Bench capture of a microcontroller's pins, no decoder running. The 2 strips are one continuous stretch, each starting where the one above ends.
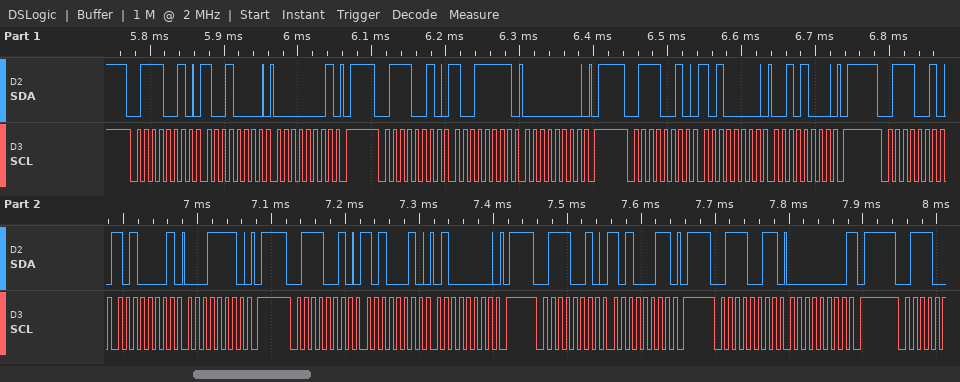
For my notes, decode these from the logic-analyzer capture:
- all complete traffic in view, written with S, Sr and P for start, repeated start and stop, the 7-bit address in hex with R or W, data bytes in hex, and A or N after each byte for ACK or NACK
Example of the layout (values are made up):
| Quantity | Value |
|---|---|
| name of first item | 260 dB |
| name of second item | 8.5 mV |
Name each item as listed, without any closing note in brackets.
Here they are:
| Quantity | Value |
|---|---|
| all complete traffic in view, written with S, Sr and P for start, repeated start and stop, the 7-bit address in hex with R or W, data bytes in hex, and A or N after each byte for ACK or NACK | S 39W A 90 A 01 A P S 39W A 9F A 00 A P S 39W A A0 A 28 A P S 39W A A1 A 1E A P S 39W A A2 A 40 A P S 39W A A3 A P S 39R A 00 N P |
